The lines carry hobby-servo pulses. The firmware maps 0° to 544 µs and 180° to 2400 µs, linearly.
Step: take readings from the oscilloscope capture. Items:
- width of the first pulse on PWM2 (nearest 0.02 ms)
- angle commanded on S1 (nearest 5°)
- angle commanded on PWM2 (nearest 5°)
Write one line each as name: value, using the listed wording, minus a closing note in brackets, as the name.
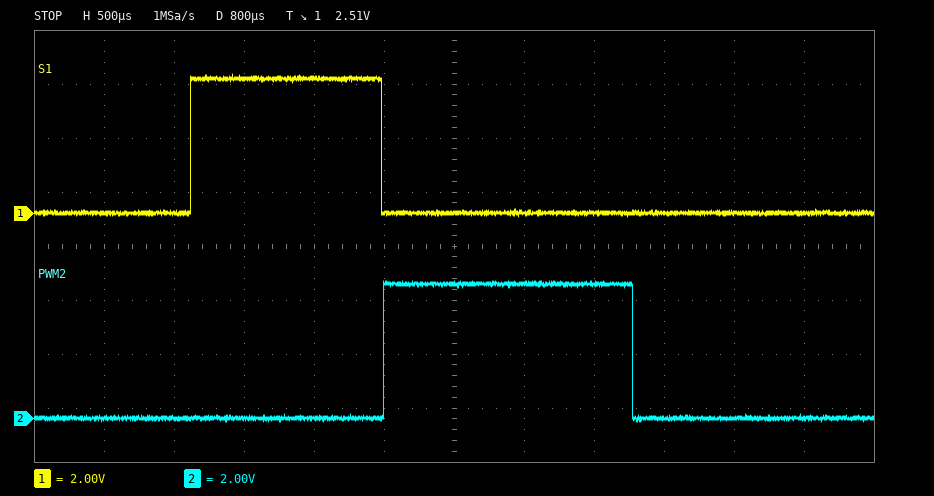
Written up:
width of the first pulse on PWM2: 1.78 ms
angle commanded on S1: 80°
angle commanded on PWM2: 120°
